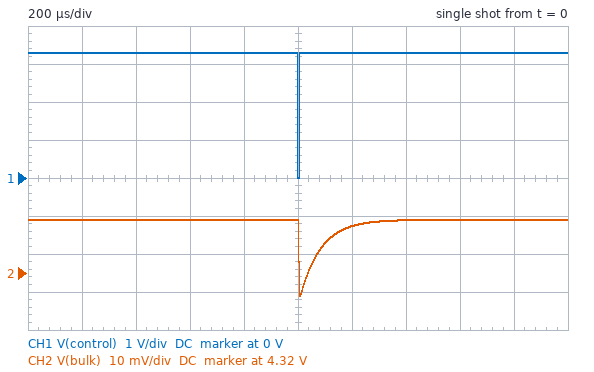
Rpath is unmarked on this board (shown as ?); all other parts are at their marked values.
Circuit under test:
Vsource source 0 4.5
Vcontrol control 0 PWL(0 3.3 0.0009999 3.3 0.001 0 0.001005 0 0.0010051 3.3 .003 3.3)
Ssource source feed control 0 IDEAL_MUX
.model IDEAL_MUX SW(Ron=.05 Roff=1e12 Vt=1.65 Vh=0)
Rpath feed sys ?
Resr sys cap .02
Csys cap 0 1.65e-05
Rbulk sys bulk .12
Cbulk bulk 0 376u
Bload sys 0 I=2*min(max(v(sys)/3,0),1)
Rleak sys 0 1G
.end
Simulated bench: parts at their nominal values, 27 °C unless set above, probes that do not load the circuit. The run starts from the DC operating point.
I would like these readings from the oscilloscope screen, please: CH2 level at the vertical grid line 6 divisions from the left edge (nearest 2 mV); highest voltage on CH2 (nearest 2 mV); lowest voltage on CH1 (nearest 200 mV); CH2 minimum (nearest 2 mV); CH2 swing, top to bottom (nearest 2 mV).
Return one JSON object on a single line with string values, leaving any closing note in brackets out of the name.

{"CH2 level at the vertical grid line 6 divisions from the left edge": "4.332 V", "highest voltage on CH2": "4.334 V", "lowest voltage on CH1": "0 V", "CH2 minimum": "4.314 V", "CH2 swing, top to bottom": "20 mV"}
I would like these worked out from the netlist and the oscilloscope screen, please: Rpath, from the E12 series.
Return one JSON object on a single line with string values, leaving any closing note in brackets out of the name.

{"Rpath, from the E12 series": "0.033 Ω"}
